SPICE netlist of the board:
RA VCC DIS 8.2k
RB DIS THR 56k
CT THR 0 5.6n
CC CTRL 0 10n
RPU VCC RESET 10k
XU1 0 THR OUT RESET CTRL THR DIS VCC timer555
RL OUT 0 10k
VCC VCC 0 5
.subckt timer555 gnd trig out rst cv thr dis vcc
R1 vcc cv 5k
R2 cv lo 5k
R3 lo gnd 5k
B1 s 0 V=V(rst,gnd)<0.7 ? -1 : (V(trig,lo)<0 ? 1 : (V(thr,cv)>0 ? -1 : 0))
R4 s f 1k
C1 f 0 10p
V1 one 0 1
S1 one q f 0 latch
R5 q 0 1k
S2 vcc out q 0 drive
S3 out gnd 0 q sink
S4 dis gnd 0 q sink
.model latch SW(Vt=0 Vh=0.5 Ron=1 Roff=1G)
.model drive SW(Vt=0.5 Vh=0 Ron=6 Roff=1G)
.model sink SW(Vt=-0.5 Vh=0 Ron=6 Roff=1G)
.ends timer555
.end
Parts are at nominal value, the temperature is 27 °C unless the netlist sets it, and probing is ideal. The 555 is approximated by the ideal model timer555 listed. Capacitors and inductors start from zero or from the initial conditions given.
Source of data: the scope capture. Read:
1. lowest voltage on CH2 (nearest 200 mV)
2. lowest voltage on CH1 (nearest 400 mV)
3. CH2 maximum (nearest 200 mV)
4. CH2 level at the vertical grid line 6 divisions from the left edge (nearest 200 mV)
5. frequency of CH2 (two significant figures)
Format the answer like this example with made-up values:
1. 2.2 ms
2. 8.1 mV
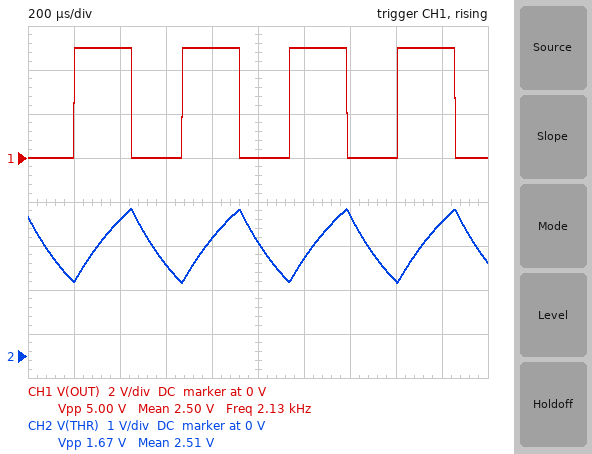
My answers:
1. 1.6 V
2. 0 V
3. 3.4 V
4. 2.2 V
5. 2.1 kHz
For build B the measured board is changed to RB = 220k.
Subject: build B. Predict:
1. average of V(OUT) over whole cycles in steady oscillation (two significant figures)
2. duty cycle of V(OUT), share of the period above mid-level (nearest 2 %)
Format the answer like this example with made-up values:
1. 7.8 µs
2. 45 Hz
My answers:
1. 2.5 V
2. 50 %
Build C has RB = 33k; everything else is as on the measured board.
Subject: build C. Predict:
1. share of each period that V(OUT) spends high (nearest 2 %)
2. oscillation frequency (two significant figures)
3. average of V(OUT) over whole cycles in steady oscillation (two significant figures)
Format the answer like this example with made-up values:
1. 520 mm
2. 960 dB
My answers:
1. 56 %
2. 3.5 kHz
3. 2.8 V
